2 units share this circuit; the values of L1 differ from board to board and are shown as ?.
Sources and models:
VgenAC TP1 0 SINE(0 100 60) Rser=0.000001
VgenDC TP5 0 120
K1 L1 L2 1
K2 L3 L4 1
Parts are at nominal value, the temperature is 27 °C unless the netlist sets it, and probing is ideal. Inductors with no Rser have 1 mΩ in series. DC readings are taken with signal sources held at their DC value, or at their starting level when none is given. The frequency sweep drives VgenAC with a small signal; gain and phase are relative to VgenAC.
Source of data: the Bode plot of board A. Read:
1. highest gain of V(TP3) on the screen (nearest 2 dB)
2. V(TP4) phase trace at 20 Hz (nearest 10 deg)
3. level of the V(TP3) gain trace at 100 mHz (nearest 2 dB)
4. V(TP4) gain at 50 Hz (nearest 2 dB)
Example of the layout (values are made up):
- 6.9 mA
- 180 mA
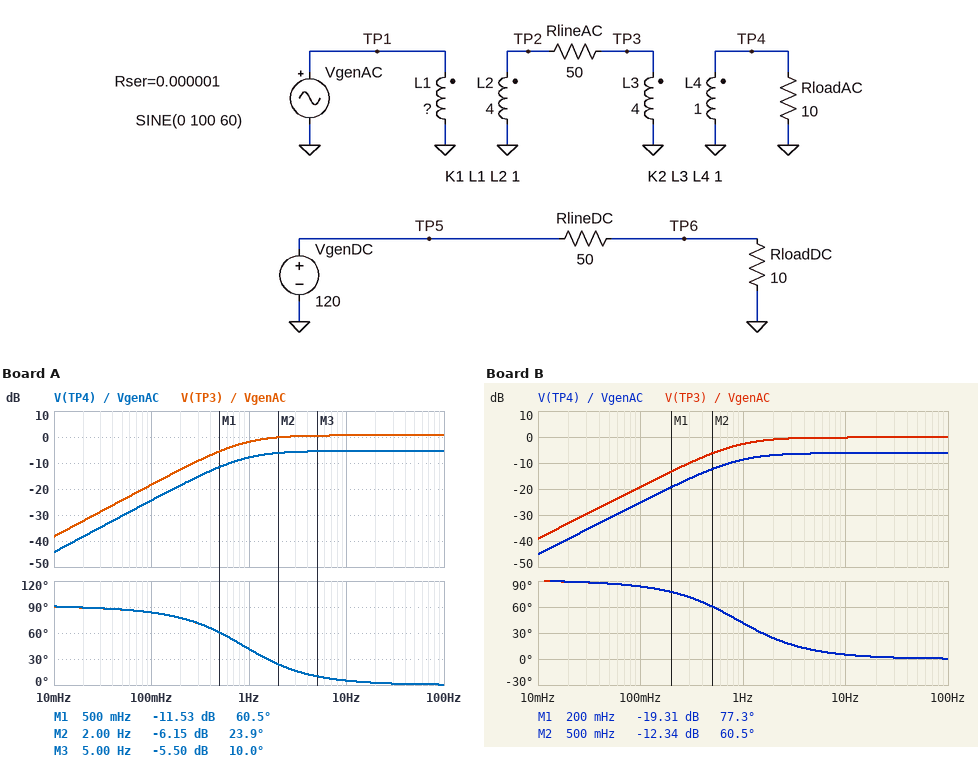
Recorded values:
- 0 dB
- 0 deg
- -18 dB
- -6 dB
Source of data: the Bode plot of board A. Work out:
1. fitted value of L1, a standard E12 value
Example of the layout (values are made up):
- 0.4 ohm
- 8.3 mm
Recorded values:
- 680 mH
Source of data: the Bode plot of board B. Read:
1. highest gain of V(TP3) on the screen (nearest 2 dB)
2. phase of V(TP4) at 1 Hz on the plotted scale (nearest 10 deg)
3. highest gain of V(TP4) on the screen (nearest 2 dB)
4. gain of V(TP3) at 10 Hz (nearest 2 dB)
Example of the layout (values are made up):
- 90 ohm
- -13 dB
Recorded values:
- 0 dB
- 40 deg
- -6 dB
- 0 dB
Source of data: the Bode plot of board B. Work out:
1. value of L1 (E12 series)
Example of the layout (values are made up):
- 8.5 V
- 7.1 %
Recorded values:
- 820 mH
